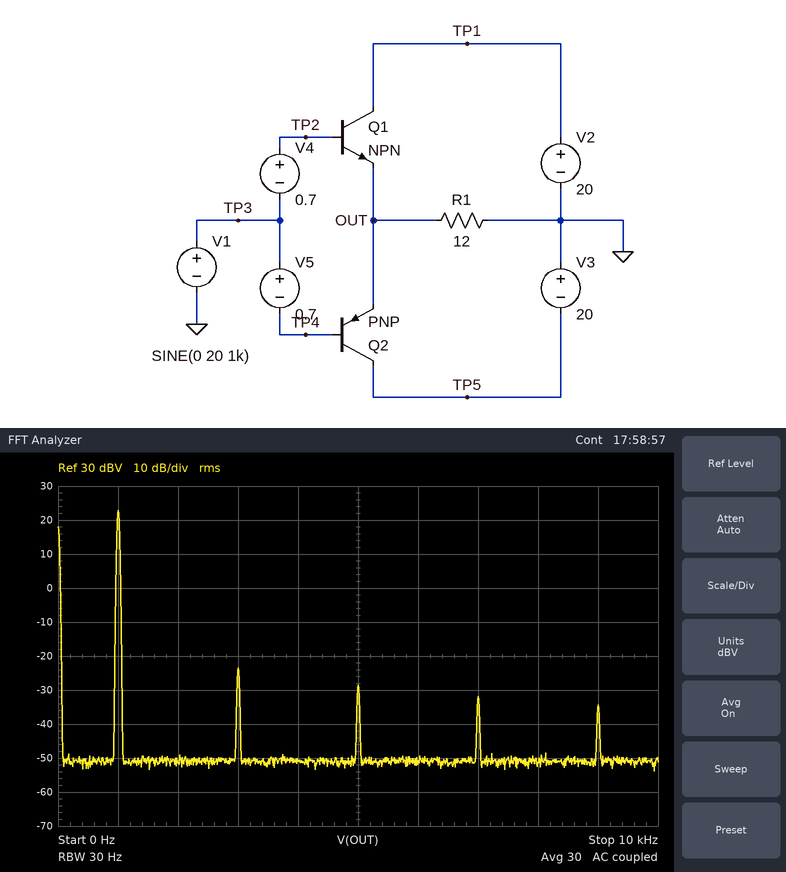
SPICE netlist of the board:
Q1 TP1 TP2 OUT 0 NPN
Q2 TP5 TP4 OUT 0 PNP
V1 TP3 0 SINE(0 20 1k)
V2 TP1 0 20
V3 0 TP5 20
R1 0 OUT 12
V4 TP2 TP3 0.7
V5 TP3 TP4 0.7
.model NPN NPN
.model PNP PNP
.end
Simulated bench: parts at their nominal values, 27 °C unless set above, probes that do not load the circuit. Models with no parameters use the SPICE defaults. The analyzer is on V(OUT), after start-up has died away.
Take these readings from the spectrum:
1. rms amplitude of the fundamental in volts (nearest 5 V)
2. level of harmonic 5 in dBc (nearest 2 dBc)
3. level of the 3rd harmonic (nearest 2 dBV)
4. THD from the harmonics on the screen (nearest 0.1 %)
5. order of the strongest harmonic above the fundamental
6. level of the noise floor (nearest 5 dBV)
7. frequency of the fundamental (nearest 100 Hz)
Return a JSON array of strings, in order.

["15 V", "-52 dBc", "-24 dBV", "0.6 %", "3", "-50 dBV", "1.0 kHz"]
